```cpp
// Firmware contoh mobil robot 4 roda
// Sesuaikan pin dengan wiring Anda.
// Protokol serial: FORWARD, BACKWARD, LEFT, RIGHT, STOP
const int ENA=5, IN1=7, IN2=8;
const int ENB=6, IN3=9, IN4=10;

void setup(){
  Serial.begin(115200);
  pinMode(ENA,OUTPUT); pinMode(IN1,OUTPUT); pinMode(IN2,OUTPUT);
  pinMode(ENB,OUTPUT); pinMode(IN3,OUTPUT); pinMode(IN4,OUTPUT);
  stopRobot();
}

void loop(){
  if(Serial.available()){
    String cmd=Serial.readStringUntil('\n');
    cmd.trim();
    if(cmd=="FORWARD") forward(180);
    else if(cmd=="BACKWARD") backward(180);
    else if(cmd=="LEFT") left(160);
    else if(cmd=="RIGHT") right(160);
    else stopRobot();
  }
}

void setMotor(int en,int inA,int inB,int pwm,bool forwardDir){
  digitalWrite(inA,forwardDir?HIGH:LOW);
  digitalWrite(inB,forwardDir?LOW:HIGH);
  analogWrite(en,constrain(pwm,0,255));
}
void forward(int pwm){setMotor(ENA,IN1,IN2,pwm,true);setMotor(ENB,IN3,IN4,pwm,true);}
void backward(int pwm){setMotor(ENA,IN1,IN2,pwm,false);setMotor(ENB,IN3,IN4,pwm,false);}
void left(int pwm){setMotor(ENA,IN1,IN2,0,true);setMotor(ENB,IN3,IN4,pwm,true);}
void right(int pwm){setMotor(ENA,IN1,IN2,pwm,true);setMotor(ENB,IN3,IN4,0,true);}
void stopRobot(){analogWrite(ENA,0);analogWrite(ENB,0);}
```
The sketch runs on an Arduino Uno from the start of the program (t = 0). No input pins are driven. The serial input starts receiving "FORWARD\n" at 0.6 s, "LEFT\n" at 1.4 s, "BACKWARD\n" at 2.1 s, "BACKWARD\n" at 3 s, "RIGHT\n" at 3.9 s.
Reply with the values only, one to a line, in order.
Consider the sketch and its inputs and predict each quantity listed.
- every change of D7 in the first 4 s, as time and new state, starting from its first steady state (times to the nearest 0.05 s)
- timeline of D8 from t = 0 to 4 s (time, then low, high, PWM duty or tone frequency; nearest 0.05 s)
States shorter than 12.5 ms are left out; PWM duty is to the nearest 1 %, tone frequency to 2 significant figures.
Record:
0 s low; 0.6 s high; 2.1 s low; 3.9 s high
0 s low; 2.1 s high; 3.9 s low
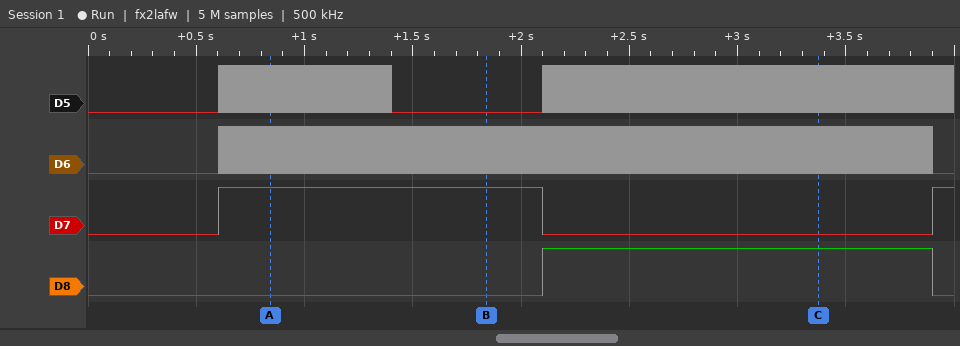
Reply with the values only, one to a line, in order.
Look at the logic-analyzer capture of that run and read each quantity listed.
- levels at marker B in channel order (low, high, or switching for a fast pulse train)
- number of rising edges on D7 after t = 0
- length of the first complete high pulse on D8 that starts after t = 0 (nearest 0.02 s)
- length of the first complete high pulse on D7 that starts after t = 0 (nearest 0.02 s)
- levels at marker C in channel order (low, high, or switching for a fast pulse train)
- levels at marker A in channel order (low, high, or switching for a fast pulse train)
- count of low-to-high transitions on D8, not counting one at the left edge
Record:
D5 low, D6 switching, D7 high, D8 low
2
1.80 s
1.50 s
D5 switching, D6 switching, D7 low, D8 high
D5 switching, D6 switching, D7 high, D8 low
1
